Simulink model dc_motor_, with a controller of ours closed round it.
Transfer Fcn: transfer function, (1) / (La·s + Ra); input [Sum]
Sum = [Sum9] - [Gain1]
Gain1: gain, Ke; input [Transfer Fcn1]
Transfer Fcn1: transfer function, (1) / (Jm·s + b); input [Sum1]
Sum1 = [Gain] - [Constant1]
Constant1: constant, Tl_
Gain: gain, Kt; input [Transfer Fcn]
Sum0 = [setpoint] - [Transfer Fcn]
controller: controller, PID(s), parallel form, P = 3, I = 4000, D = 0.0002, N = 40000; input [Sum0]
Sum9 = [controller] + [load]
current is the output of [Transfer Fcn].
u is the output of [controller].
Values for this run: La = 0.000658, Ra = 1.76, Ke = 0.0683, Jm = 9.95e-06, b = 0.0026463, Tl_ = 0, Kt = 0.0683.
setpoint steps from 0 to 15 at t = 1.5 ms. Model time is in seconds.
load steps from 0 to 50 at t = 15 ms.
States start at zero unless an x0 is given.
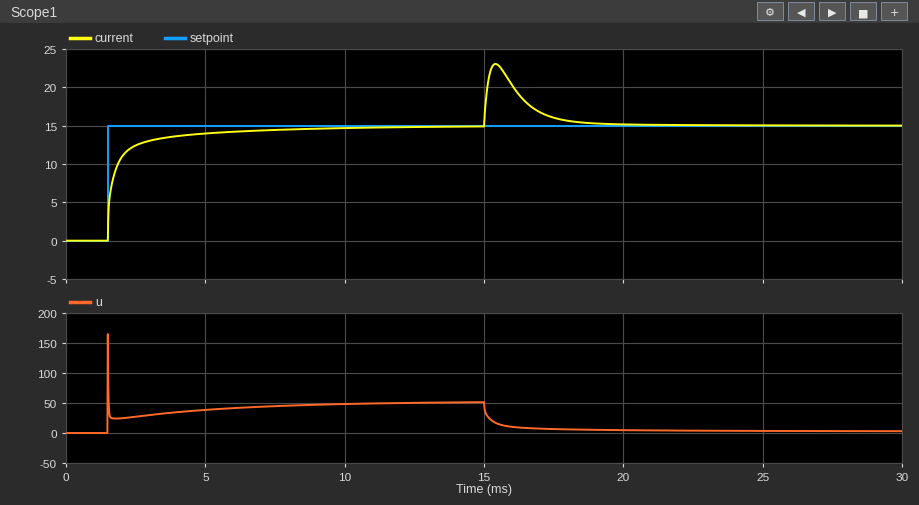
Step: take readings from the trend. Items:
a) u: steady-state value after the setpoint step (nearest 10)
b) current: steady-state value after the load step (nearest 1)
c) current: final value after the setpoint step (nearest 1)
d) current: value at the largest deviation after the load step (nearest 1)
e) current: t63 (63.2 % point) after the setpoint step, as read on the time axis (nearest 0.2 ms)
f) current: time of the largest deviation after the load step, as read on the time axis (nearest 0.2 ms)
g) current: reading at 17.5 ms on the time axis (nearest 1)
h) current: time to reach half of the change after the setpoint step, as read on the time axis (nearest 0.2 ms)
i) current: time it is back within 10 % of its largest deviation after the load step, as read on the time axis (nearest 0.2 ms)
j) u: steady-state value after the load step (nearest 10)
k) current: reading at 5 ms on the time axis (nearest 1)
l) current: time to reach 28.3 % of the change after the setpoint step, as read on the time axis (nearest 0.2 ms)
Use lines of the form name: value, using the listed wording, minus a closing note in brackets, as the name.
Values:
u: steady-state value after the setpoint step: 50
current: steady-state value after the load step: 15
current: final value after the setpoint step: 15
current: value at the largest deviation after the load step: 23
current: t63 (63.2 % point) after the setpoint step, as read on the time axis: 1.8 ms
current: time of the largest deviation after the load step, as read on the time axis: 15.4 ms
current: reading at 17.5 ms on the time axis: 16
current: time to reach half of the change after the setpoint step, as read on the time axis: 1.6 ms
current: time it is back within 10 % of its largest deviation after the load step, as read on the time axis: 17.8 ms
u: steady-state value after the load step: 0
current: reading at 5 ms on the time axis: 14
current: time to reach 28.3 % of the change after the setpoint step, as read on the time axis: 1.6 ms
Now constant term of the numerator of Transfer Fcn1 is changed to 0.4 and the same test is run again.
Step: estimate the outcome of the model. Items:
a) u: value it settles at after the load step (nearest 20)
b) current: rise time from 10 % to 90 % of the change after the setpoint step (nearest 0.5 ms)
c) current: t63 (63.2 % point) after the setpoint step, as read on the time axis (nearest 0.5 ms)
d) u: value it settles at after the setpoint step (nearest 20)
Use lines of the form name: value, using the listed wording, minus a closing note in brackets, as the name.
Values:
u: value it settles at after the load step: -20
current: rise time from 10 % to 90 % of the change after the setpoint step: 1.5 ms
current: t63 (63.2 % point) after the setpoint step, as read on the time axis: 2.0 ms
u: value it settles at after the setpoint step: 40
